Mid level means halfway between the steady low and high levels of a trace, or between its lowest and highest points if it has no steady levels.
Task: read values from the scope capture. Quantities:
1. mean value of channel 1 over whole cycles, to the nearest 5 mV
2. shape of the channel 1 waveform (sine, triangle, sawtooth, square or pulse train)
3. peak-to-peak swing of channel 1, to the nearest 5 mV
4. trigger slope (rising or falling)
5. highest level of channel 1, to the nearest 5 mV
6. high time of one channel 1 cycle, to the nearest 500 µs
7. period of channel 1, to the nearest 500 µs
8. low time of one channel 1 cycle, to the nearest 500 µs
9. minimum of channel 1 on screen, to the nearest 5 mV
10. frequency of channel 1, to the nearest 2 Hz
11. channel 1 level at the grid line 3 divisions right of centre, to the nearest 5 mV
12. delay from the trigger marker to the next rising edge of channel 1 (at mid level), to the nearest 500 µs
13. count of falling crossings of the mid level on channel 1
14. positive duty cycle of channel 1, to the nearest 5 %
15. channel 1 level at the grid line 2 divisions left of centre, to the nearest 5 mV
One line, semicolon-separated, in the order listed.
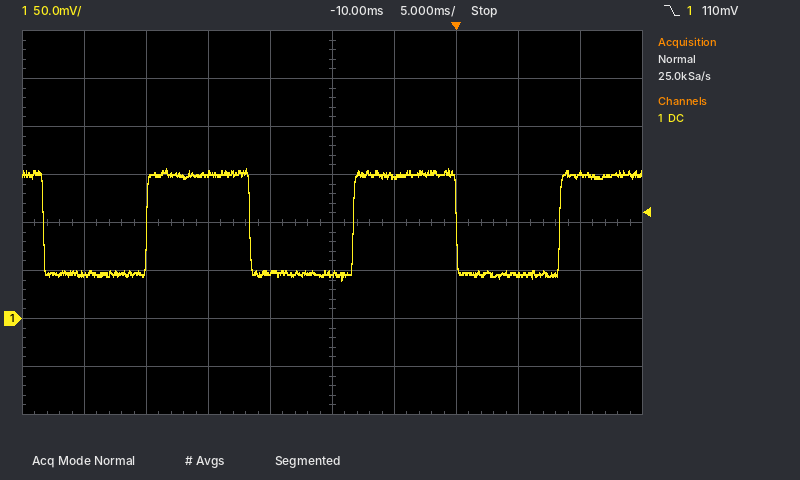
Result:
100 mV; square; 115 mV; falling; 155 mV; 8.5 ms; 16.5 ms; 8.5 ms; 40 mV; 60 Hz; 45 mV; 8.5 ms; 3; 50 %; 150 mV
